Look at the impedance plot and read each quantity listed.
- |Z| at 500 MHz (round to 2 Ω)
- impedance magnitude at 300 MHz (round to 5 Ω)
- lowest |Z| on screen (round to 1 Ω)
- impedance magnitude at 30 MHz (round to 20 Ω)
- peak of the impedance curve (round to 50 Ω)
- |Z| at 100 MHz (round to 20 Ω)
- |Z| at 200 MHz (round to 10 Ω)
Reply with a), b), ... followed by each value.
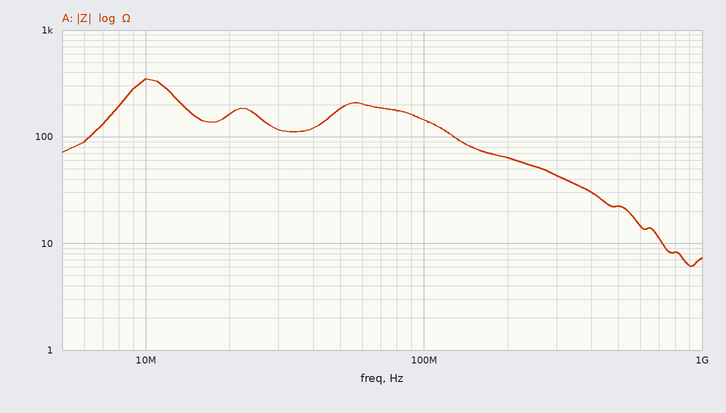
a) 22 Ω
b) 45 Ω
c) 6 Ω
d) 120 Ω
e) 350 Ω
f) 140 Ω
g) 60 Ω
